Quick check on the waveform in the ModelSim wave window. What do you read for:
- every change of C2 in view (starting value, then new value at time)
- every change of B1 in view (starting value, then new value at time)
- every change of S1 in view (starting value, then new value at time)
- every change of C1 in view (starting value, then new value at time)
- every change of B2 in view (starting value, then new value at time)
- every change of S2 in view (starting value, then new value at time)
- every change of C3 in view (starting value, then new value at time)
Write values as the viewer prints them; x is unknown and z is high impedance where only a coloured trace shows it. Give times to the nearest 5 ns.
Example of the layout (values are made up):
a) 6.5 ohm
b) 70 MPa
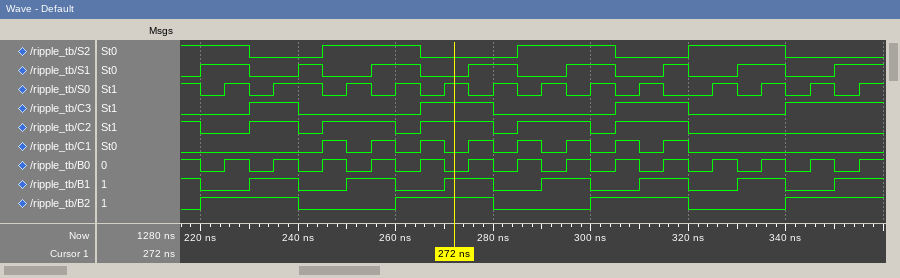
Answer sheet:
a) 1, 0 at 220 ns, 1 at 230 ns, 0 at 240 ns, 1 at 245 ns, 0 at 260 ns, 1 at 265 ns, 0 at 280 ns, 1 at 285 ns, 0 at 300 ns, 1 at 305 ns, 0 at 320 ns
b) 1, 0 at 220 ns, 1 at 230 ns, 0 at 240 ns, 1 at 250 ns, 0 at 260 ns, 1 at 270 ns, 0 at 280 ns, 1 at 290 ns, 0 at 300 ns, 1 at 310 ns, 0 at 320 ns, 1 at 330 ns, 0 at 340 ns, 1 at 350 ns
c) 0, 1 at 220 ns, 0 at 230 ns, 1 at 240 ns, 0 at 245 ns, 1 at 255 ns, 0 at 265 ns, 1 at 275 ns, 0 at 285 ns, 1 at 295 ns, 0 at 305 ns, 1 at 315 ns, 0 at 320 ns, 1 at 330 ns, 0 at 340 ns, 1 at 350 ns
d) 0, 1 at 245 ns, 0 at 250 ns, 1 at 255 ns, 0 at 260 ns, 1 at 265 ns, 0 at 270 ns, 1 at 275 ns, 0 at 280 ns, 1 at 285 ns, 0 at 290 ns, 1 at 295 ns, 0 at 300 ns, 1 at 305 ns, 0 at 310 ns, 1 at 315 ns, 0 at 320 ns
e) 0, 1 at 220 ns, 0 at 240 ns, 1 at 260 ns, 0 at 280 ns, 1 at 300 ns, 0 at 320 ns, 1 at 340 ns
f) 1, 0 at 230 ns, 1 at 245 ns, 0 at 265 ns, 1 at 285 ns, 0 at 305 ns, 1 at 320 ns, 0 at 340 ns
g) 0, 1 at 230 ns, 0 at 240 ns, 1 at 265 ns, 0 at 280 ns, 1 at 305 ns, 0 at 320 ns, 1 at 340 ns
